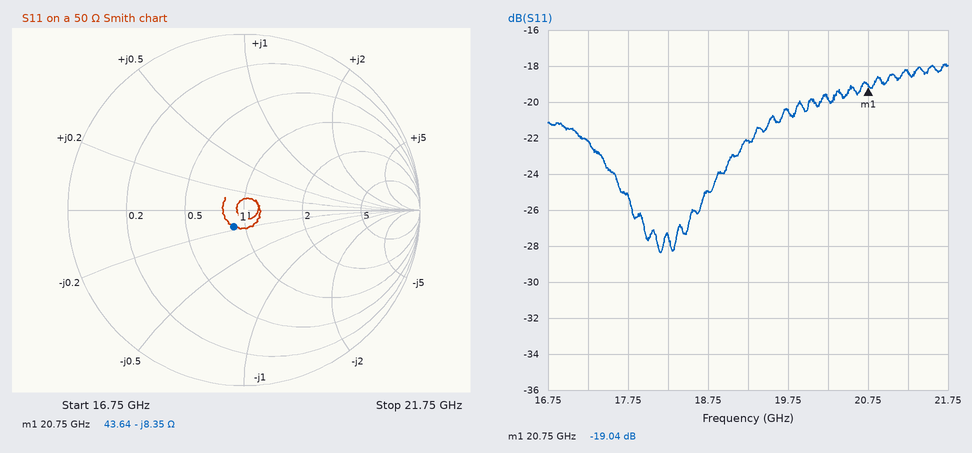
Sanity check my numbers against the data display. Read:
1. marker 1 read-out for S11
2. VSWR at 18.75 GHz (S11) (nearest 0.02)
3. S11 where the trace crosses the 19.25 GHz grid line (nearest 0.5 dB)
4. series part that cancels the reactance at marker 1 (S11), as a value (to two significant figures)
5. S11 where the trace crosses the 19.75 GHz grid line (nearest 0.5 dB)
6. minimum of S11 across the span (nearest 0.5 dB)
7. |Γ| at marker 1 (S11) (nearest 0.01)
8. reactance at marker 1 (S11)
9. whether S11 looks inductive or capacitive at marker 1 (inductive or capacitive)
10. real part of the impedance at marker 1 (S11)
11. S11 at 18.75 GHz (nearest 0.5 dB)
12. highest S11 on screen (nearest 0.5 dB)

-19.04 dB
1.12
-22.0 dB
64 pH
-20.5 dB
-28.5 dB
0.11
-8.35 Ω
capacitive
43.64 Ω
-25.0 dB
-18.0 dB
